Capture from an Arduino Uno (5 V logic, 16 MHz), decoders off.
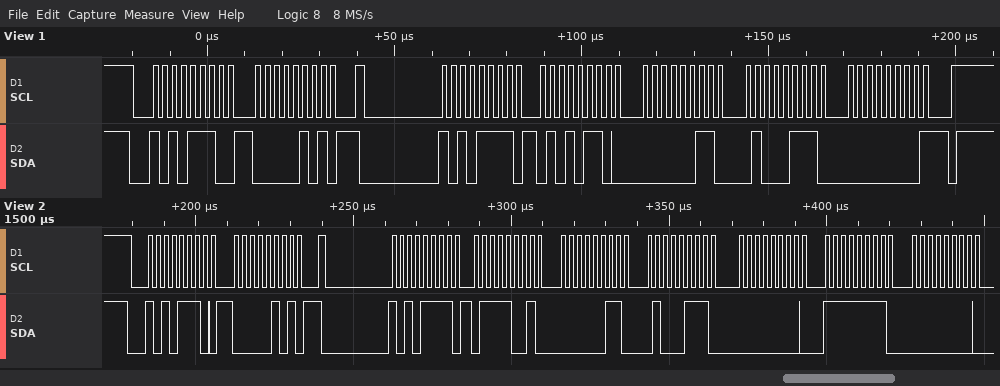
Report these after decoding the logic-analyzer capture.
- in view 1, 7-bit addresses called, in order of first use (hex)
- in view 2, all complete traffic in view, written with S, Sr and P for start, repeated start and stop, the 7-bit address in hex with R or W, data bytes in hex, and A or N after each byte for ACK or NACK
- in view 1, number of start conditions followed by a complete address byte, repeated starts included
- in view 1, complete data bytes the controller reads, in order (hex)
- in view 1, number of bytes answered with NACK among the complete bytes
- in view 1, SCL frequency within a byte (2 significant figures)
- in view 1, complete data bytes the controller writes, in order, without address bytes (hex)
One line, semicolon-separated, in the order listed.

0x57; S 57W A 05 A Sr 57R A 79 A 03 A 47 A 00 A FF A 00 A; 2; 56 03 47 00; 1; 400 kHz; 05
